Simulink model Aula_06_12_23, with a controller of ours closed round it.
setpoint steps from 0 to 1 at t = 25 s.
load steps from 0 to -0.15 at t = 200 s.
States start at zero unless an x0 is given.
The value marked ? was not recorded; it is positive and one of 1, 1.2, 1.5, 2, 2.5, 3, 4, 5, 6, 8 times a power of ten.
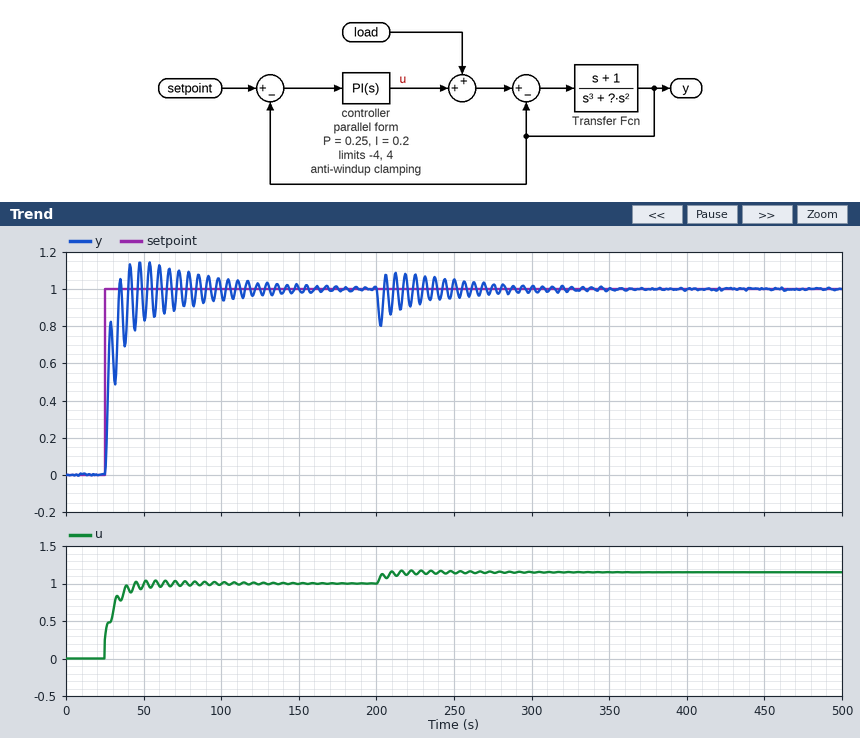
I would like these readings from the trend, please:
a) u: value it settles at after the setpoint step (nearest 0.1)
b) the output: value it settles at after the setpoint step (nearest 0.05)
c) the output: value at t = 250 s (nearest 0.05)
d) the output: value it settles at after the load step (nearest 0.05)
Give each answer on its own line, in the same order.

1.0
1.00
1.05
1.00
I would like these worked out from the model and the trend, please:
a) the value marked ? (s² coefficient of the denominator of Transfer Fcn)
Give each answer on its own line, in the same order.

1.5
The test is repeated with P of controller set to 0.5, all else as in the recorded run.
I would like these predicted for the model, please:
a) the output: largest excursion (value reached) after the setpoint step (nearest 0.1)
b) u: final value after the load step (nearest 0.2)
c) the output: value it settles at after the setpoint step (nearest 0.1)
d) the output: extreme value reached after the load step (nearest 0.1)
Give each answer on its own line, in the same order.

1.1
1.2
1.0
0.8
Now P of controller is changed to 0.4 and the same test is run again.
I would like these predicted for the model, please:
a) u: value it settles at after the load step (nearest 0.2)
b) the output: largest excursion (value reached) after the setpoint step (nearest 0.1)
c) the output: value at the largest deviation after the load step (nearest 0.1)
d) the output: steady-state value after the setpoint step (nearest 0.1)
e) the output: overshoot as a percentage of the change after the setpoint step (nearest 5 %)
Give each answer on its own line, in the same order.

1.2
1.1
0.8
1.0
10 %
